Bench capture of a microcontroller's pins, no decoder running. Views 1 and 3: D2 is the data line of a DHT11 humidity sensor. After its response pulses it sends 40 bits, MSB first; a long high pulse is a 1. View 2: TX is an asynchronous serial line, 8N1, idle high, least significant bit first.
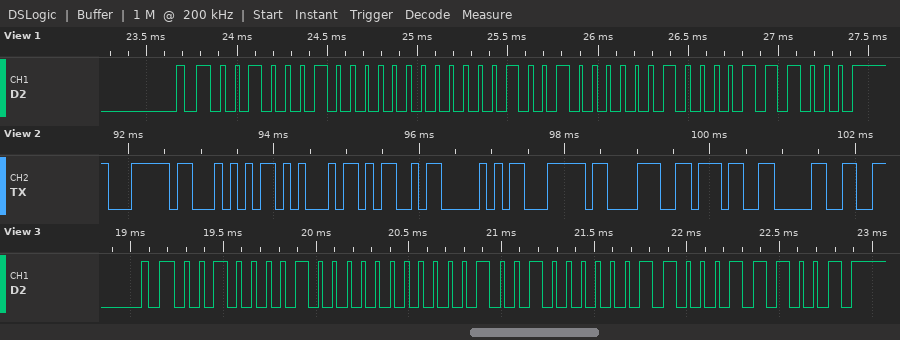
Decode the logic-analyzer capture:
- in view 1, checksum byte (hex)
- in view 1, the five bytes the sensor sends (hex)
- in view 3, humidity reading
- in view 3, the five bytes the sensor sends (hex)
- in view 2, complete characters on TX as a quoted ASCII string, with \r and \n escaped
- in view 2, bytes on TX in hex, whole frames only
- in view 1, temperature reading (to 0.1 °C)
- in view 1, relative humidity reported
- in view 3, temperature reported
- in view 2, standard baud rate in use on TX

0x38
22 00 12 04 38
33 %
21 00 12 06 39
"|TEMP|870"
7C 54 45 4D 50 7C 38 37 30
18.4 °C
34 %
18.6 °C
9600 baud
